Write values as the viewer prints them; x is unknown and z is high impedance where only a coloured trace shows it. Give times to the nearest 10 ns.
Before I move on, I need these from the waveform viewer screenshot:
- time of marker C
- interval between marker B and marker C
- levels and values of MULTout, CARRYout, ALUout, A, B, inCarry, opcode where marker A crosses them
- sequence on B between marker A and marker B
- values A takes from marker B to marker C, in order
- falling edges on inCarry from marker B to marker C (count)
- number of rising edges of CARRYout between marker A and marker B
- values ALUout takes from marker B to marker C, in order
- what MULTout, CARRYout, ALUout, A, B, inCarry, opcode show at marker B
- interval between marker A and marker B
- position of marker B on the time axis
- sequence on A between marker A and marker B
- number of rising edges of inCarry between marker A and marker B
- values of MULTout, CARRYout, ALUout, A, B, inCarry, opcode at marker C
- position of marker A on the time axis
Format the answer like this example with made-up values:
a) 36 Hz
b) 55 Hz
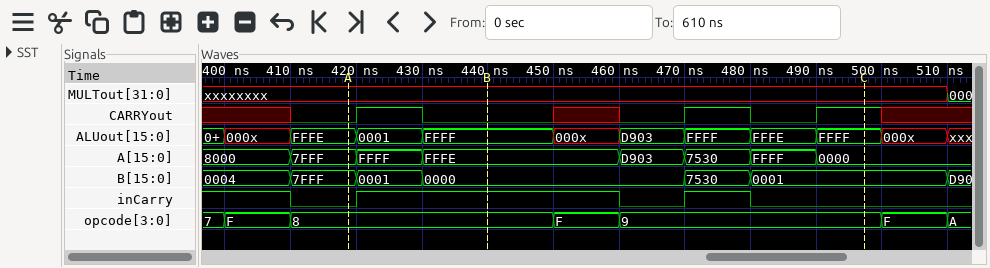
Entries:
a) 500 ns
b) 60 ns
c) MULTout=xxxxxxxx, CARRYout=0, ALUout=FFFE, A=7FFF, B=7FFF, inCarry=0, opcode=8
d) 7FFF, 0001, 0000
e) FFFE, D903, 7530, FFFF, 0000
f) 2
g) 1
h) FFFF, 000x, D903, FFFF, FFFE, FFFF
i) MULTout=xxxxxxxx, CARRYout=0, ALUout=FFFF, A=FFFE, B=0000, inCarry=1, opcode=8
j) 20 ns
k) 440 ns
l) 7FFF, FFFF, FFFE
m) 1
n) MULTout=xxxxxxxx, CARRYout=1, ALUout=FFFF, A=0000, B=0001, inCarry=0, opcode=9
o) 420 ns
